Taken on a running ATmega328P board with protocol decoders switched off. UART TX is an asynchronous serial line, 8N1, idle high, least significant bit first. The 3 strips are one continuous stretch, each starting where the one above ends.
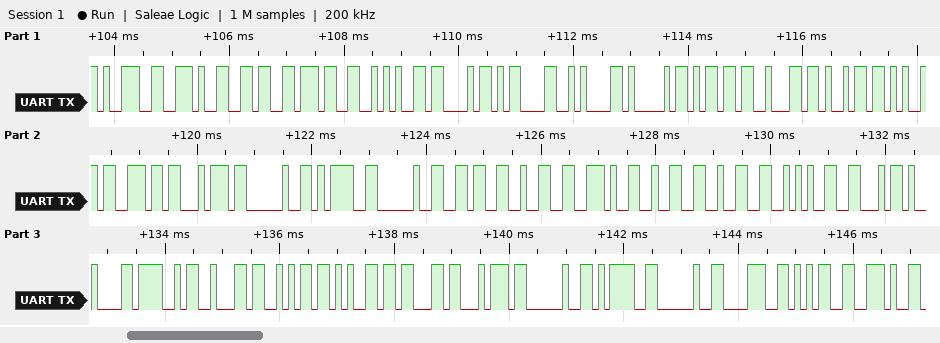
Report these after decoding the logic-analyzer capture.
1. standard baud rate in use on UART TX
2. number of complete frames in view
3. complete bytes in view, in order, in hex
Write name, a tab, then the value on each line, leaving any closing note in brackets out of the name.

standard baud rate in use on UART TX	9600 baud
number of complete frames in view	38
complete bytes in view, in order, in hex	39 2E 36 37 2A 43 0D 0A 41 6D 62 69 65 6E 74 20 3D 20 36 32 2E 32 32 2A 46 09 4F 62 6A 65 63 74 20 3D 20 38 35 2E
